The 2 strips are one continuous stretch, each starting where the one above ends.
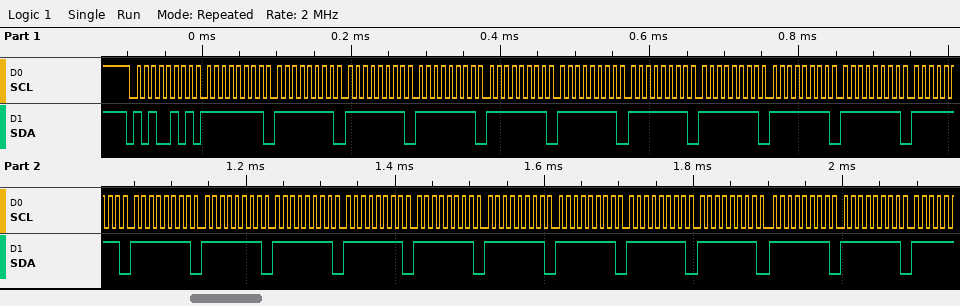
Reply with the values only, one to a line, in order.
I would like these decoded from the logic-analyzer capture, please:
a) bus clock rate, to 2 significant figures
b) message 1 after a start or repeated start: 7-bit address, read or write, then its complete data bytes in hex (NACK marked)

100 kHz
0x52 read: FF FF FF FF FF FF FF FF FF FF FF FF FF FF FF FF FF FF FF FF FF FF
